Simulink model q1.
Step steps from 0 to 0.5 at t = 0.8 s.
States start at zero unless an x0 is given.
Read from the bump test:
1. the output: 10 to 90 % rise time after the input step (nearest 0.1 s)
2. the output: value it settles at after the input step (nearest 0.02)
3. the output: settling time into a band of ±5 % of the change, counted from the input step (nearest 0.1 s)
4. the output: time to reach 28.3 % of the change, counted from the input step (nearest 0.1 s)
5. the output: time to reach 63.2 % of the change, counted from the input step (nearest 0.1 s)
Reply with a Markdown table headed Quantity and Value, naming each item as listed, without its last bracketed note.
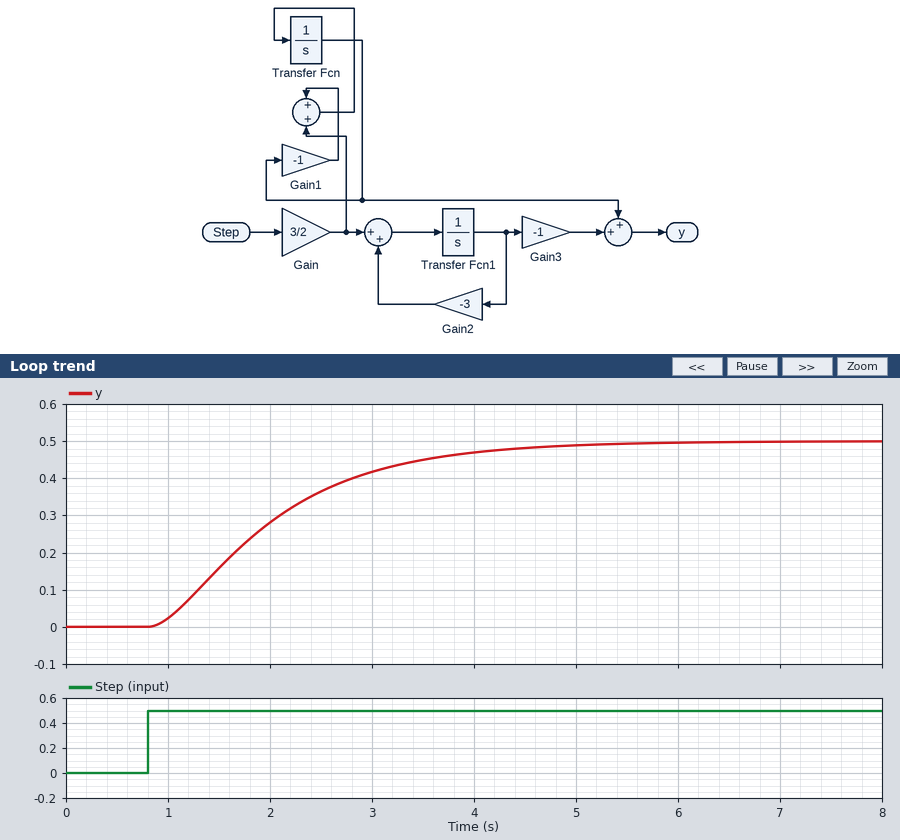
| Quantity | Value |
|---|---|
| the output: 10 to 90 % rise time after the input step | 2.4 s |
| the output: value it settles at after the input step | 0.50 |
| the output: settling time into a band of ±5 % of the change, counted from the input step | 3.4 s |
| the output: time to reach 28.3 % of the change, counted from the input step | 0.6 s |
| the output: time to reach 63.2 % of the change, counted from the input step | 1.4 s |
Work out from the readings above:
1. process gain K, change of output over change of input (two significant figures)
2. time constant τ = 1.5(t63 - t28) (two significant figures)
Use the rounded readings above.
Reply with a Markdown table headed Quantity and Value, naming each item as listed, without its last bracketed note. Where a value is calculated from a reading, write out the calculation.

| Quantity | Value |
|---|---|
| process gain K, change of output over change of input | (0.5 - 0) / 0.5 = 1.0 |
| time constant τ = 1.5(t63 - t28) | 1.5 × (1.4 - 0.6) = 1.2 s |
